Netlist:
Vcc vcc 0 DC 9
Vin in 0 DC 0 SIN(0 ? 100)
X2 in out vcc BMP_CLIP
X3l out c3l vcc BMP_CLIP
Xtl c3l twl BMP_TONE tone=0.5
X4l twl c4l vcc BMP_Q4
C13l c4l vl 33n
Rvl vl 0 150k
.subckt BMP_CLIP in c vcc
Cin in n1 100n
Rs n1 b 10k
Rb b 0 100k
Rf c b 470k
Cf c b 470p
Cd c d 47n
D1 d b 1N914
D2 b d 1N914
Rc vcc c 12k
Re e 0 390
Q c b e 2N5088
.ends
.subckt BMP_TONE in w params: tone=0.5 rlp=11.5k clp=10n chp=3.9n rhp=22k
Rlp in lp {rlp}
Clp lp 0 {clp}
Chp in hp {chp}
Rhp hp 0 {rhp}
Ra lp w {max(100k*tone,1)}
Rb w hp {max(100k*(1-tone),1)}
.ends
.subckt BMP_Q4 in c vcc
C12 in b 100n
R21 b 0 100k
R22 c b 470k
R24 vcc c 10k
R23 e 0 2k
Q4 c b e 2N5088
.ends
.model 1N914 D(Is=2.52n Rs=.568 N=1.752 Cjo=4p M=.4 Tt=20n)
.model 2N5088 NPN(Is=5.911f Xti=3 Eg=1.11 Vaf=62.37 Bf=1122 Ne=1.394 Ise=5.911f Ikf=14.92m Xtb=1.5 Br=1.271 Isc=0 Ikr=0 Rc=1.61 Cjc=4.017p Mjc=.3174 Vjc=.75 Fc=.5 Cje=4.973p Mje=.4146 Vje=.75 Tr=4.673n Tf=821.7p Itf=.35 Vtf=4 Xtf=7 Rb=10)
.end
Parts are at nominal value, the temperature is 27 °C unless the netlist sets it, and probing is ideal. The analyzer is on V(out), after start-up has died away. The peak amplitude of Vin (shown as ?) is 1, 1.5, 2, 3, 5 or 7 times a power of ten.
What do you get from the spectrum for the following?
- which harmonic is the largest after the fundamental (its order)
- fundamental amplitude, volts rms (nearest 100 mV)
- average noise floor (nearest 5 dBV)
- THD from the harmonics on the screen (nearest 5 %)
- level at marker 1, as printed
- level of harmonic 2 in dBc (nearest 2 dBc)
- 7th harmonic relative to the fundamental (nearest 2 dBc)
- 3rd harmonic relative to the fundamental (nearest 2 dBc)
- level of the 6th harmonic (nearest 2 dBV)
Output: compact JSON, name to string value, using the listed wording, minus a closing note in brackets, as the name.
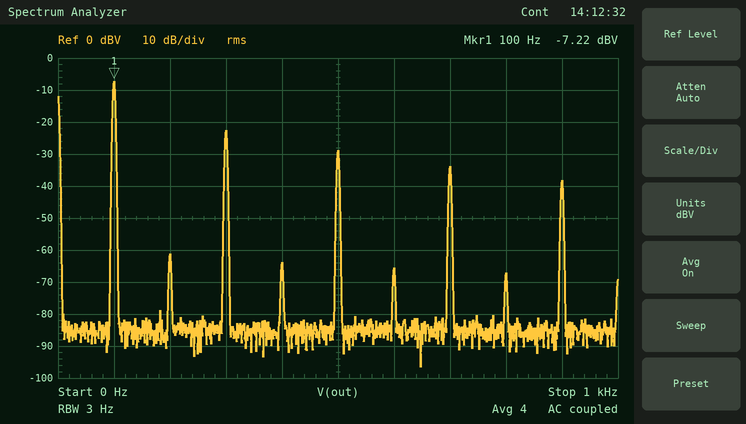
{"which harmonic is the largest after the fundamental": "3", "fundamental amplitude, volts rms": "400 mV", "average noise floor": "-85 dBV", "THD from the harmonics on the screen": "20 %", "level at marker 1, as printed": "-7.22 dBV", "level of harmonic 2 in dBc": "-54 dBc", "7th harmonic relative to the fundamental": "-26 dBc", "3rd harmonic relative to the fundamental": "-16 dBc", "level of the 6th harmonic": "-66 dBV"}
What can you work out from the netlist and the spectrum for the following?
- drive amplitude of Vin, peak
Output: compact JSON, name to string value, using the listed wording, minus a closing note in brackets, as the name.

{"drive amplitude of Vin, peak": "300 mV"}
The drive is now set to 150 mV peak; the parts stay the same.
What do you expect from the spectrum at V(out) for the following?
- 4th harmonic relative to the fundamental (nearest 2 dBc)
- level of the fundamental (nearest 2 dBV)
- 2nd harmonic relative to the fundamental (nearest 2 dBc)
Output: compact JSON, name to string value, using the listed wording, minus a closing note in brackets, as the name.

{"4th harmonic relative to the fundamental": "-58 dBc", "level of the fundamental": "-10 dBV", "2nd harmonic relative to the fundamental": "-56 dBc"}
